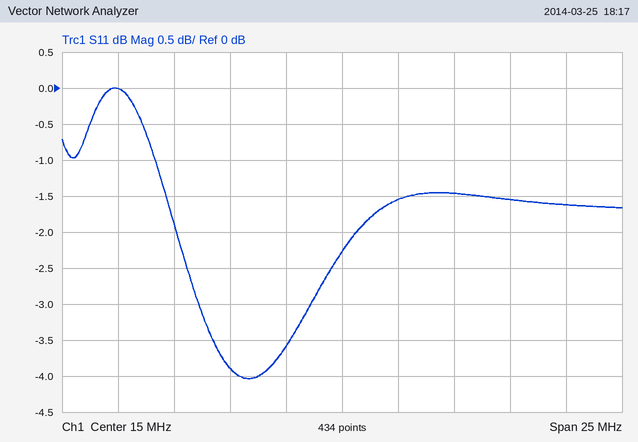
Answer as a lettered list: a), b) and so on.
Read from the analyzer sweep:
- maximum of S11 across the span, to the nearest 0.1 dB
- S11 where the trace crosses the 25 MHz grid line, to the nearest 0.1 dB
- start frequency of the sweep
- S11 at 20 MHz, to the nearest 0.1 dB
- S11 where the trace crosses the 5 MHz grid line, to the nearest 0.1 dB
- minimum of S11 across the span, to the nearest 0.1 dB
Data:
a) 0.0 dB
b) -1.6 dB
c) 2.5 MHz
d) -1.5 dB
e) 0.0 dB
f) -4.0 dB
